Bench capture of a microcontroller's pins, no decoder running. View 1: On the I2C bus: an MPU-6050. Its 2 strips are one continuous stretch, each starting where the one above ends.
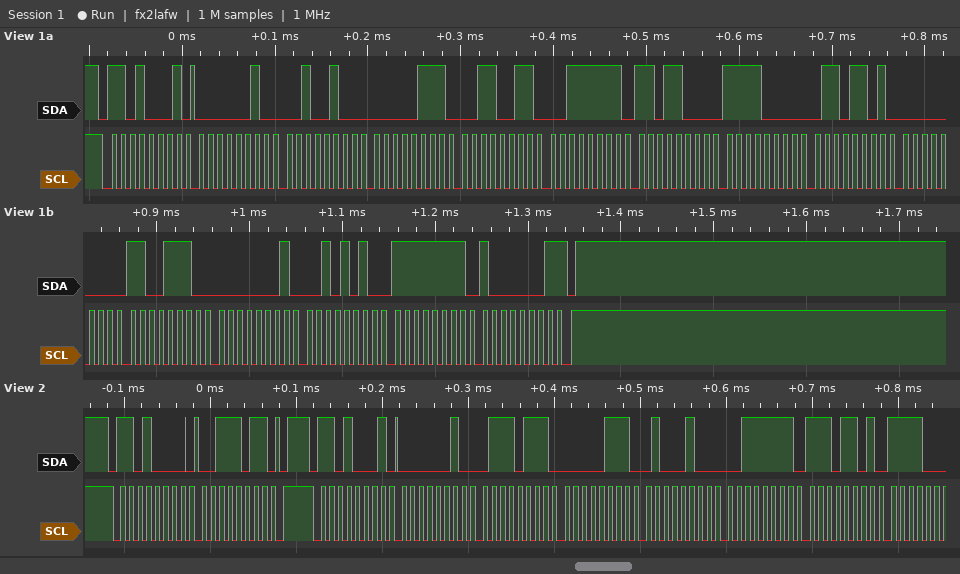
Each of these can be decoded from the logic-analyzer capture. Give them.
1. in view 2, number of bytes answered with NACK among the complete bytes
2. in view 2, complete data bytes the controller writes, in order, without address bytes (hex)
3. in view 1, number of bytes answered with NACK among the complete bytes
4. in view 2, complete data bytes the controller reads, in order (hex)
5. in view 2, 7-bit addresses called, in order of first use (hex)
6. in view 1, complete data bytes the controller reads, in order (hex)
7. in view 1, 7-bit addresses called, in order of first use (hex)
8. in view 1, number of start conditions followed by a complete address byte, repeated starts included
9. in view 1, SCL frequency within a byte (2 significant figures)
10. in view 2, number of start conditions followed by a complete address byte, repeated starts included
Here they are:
0
3B
1
02 77 07 44 3F ED
0x68
02 24 07 33 3F D8 F0 6D 00 CE 01 2A FF 81
0x68
1
100 kHz
2
